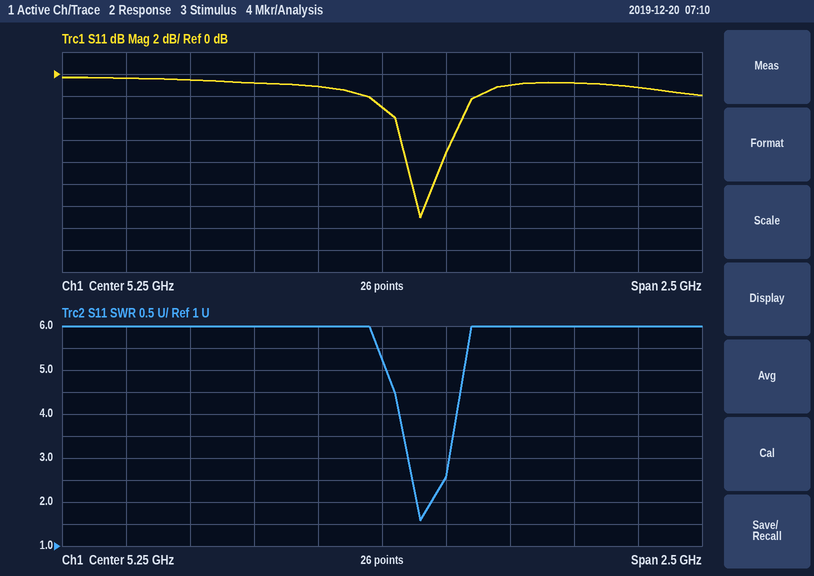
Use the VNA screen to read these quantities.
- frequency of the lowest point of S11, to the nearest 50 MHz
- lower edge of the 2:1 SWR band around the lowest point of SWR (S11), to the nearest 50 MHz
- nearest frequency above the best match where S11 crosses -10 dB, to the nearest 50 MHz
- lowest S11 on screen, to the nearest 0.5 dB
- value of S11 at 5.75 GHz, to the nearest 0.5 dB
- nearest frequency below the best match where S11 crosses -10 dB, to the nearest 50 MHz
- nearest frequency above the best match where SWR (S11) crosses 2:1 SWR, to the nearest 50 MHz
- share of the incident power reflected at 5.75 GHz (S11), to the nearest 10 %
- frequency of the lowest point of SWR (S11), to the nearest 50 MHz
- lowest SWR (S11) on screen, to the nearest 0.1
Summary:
5.40 GHz
5.40 GHz
5.45 GHz
-13.0 dB
-1.0 dB
5.35 GHz
5.45 GHz
80 %
5.40 GHz
1.6
